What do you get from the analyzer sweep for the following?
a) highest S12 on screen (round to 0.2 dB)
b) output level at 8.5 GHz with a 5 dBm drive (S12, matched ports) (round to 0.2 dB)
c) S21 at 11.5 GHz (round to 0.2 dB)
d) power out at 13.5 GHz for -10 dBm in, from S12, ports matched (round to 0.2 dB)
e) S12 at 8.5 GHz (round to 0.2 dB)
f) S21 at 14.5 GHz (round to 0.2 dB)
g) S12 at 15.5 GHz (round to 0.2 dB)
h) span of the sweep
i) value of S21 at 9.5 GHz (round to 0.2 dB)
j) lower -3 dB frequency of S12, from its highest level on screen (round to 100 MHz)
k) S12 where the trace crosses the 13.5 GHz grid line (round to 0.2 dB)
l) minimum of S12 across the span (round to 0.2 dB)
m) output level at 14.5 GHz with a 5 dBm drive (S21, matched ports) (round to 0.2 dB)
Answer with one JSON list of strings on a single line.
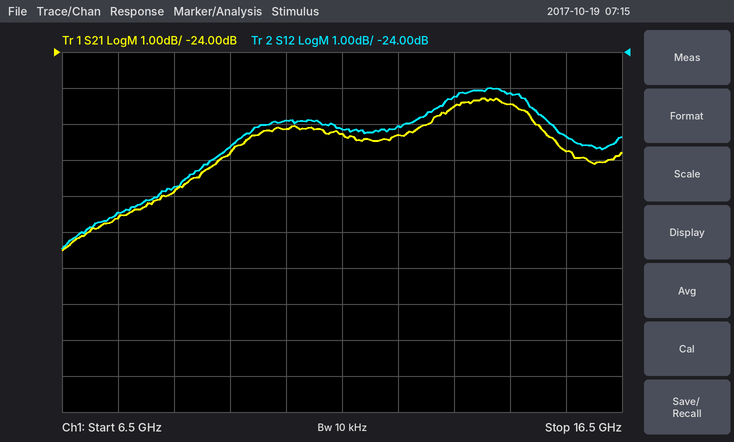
["-25.0 dB", "-22.8 dBm", "-26.2 dB", "-35.2 dBm", "-27.8 dB", "-25.4 dB", "-26.4 dB", "10 GHz", "-26.8 dB", "8.2 GHz", "-25.2 dB", "-29.4 dB", "-20.4 dBm"]
